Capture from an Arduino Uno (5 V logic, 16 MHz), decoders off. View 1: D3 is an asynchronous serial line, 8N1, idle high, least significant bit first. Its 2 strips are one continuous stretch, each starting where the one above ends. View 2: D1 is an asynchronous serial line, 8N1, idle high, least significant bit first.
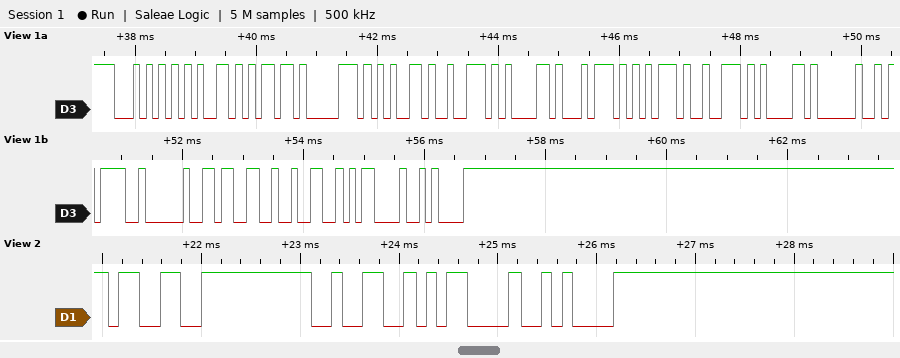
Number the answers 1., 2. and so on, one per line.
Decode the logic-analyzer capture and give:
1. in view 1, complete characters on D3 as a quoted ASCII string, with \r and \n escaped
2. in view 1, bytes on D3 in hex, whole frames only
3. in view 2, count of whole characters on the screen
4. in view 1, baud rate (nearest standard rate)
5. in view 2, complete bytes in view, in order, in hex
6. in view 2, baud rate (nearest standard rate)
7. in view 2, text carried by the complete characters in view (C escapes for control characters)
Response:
1. "Temperatura = 32\r\n"
2. 54 65 6D 70 65 72 61 74 75 72 61 20 3D 20 33 32 0D 0A
3. 4
4. 9600 baud
5. 33 32 0D 0A
6. 9600 baud
7. "32\r\n"
